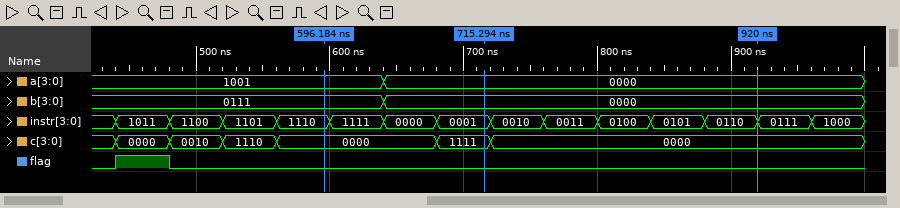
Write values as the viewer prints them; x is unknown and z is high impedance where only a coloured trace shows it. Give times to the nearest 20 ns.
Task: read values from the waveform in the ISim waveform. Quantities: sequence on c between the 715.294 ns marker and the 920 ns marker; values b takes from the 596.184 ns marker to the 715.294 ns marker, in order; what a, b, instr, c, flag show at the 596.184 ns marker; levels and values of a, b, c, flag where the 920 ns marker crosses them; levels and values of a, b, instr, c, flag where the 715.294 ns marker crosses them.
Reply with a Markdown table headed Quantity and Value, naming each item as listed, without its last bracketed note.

| Quantity | Value |
|---|---|
| sequence on c between the 715.294 ns marker and the 920 ns marker | 1111, 0000 |
| values b takes from the 596.184 ns marker to the 715.294 ns marker, in order | 0111, 0000 |
| what a, b, instr, c, flag show at the 596.184 ns marker | a=1001, b=0111, instr=1110, c=0000, flag=0 |
| levels and values of a, b, c, flag where the 920 ns marker crosses them | a=0000, b=0000, c=0000, flag=0 |
| levels and values of a, b, instr, c, flag where the 715.294 ns marker crosses them | a=0000, b=0000, instr=0001, c=1111, flag=0 |
